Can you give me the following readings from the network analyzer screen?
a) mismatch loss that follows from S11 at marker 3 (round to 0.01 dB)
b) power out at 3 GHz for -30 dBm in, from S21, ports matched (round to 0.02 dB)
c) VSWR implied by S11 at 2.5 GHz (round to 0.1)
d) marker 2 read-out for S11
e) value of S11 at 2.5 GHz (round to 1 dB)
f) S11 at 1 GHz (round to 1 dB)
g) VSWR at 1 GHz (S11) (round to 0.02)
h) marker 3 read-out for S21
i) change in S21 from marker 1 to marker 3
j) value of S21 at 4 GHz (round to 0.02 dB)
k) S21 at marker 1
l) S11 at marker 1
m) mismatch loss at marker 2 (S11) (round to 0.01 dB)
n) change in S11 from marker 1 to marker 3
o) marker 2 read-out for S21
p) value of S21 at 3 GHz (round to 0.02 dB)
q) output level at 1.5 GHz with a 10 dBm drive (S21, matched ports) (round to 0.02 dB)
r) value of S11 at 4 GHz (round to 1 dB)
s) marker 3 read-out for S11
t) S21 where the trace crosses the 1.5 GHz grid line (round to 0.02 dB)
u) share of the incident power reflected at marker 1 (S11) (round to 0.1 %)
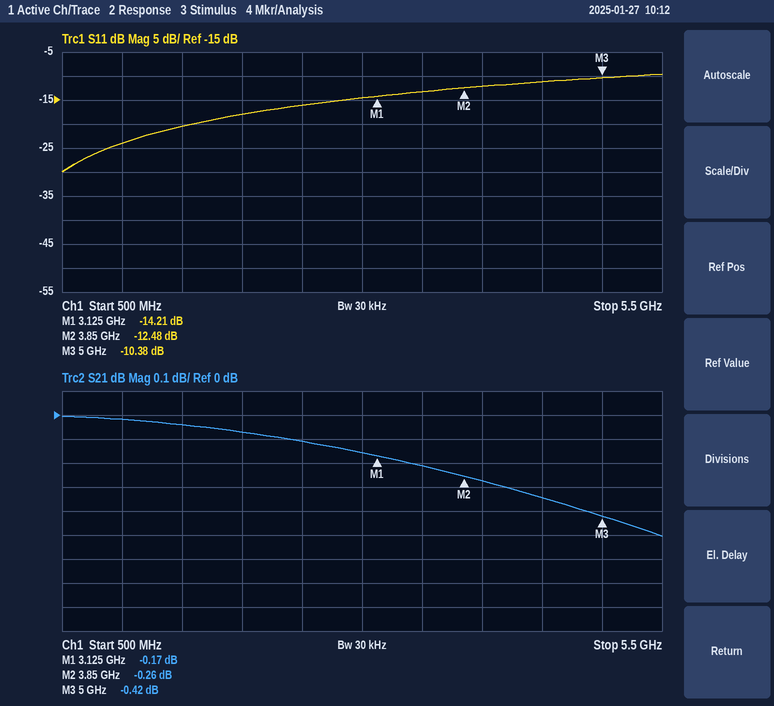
0.42 dB
-30.16 dBm
1.4
-12.48 dB
-16 dB
-24 dB
1.14
-0.42 dB
-0.25 dB
-0.28 dB
-0.17 dB
-14.21 dB
0.25 dB
3.83 dB
-0.26 dB
-0.16 dB
9.96 dBm
-12 dB
-10.38 dB
-0.04 dB
3.8 %
